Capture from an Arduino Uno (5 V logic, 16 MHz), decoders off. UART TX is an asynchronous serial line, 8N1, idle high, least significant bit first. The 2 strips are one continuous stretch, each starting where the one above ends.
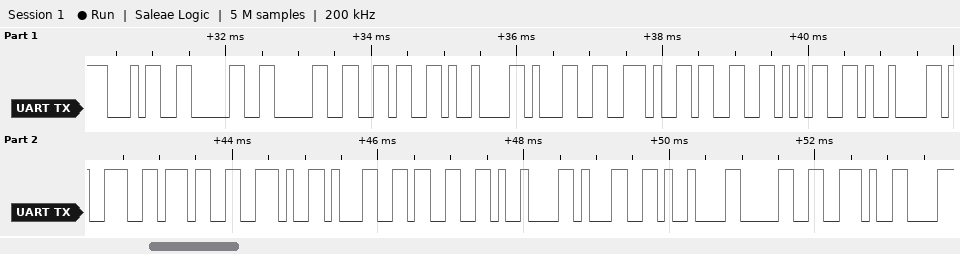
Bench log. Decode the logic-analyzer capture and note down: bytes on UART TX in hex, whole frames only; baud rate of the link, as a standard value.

0x34 0x30 0x30 0x36 0x09 0x31 0x2E 0x33 0x35 0x09 0x39 0x37 0x2E 0x31 0x33 0x09 0x31 0x09 0x30 0x2E
9600 baud
